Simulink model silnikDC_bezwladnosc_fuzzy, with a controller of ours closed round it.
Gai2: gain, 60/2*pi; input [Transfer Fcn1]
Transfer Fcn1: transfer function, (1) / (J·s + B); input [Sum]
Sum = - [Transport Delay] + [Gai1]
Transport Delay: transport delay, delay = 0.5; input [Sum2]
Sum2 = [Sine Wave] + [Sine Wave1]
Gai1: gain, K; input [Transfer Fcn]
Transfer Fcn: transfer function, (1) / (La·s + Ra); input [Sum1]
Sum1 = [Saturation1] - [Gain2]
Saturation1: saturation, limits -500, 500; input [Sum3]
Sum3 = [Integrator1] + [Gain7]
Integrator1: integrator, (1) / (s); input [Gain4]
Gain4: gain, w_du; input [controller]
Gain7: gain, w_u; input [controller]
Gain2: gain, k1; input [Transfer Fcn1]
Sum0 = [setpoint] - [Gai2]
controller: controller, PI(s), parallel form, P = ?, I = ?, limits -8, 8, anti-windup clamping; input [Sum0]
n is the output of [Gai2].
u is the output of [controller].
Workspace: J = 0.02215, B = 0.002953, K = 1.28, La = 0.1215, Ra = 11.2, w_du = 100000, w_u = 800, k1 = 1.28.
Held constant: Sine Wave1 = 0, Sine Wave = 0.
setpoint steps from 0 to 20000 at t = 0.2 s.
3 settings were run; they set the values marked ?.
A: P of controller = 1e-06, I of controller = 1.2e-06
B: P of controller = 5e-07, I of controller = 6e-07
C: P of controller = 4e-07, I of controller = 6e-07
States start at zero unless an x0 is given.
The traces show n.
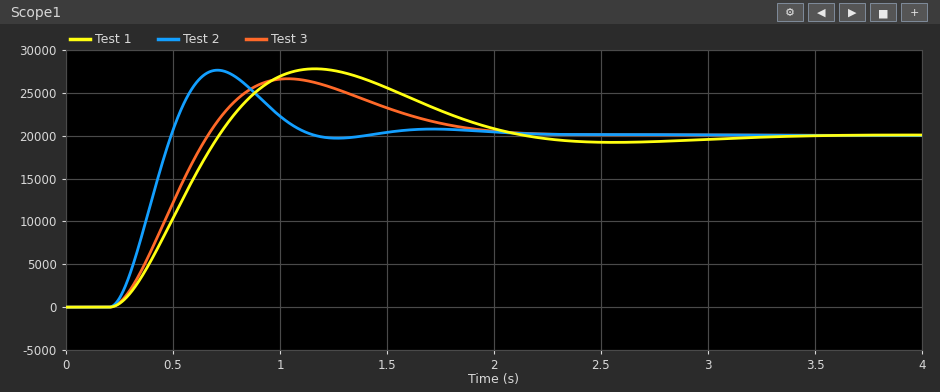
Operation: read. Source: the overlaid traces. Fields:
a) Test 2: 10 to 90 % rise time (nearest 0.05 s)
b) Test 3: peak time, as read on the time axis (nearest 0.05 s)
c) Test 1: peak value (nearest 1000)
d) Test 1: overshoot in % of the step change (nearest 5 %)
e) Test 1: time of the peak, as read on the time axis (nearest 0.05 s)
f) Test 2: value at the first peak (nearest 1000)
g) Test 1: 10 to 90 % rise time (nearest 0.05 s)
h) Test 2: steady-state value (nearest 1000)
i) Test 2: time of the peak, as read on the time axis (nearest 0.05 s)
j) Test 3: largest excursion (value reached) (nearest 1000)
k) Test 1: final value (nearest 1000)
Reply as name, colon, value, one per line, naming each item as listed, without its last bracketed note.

Test 2: 10 to 90 % rise time: 0.20 s
Test 3: peak time, as read on the time axis: 1.05 s
Test 1: peak value: 28000
Test 1: overshoot in % of the step change: 40 %
Test 1: time of the peak, as read on the time axis: 1.15 s
Test 2: value at the first peak: 28000
Test 1: 10 to 90 % rise time: 0.35 s
Test 2: steady-state value: 20000
Test 2: time of the peak, as read on the time axis: 0.70 s
Test 3: largest excursion (value reached): 27000
Test 1: final value: 20000
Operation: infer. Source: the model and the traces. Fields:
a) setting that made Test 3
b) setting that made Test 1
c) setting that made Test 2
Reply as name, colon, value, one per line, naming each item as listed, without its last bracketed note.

setting that made Test 3: B
setting that made Test 1: C
setting that made Test 2: A
